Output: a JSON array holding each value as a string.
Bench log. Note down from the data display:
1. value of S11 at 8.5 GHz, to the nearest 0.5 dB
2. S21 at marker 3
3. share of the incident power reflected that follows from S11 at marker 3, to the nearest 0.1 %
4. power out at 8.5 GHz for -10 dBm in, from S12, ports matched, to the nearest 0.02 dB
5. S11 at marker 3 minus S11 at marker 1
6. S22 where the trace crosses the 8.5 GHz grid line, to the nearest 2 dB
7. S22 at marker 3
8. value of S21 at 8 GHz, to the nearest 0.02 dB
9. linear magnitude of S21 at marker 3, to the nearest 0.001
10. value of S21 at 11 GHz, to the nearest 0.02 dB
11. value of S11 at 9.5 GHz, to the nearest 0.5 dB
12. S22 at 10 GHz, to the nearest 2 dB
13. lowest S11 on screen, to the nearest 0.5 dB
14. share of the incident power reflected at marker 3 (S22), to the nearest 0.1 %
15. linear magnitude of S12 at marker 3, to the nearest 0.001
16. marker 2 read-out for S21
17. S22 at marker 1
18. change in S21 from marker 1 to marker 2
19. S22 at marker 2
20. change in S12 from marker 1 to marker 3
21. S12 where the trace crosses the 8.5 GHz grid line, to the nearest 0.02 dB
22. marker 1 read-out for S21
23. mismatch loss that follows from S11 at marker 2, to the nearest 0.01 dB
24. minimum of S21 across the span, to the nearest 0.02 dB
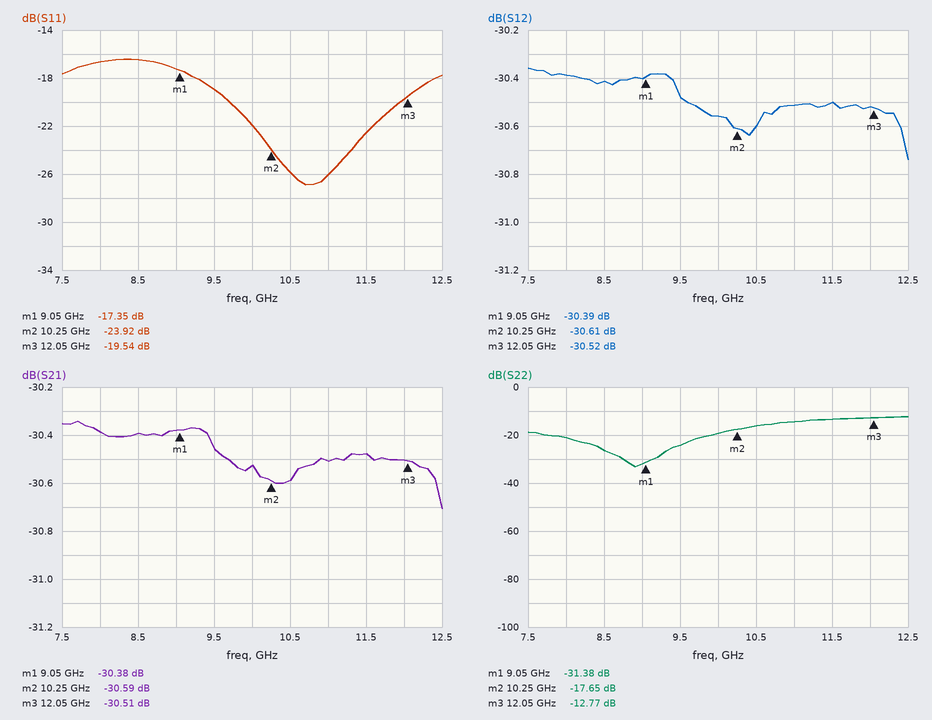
["-16.5 dB", "-30.51 dB", "1.1 %", "-40.42 dBm", "-2.19 dB", "-26 dB", "-12.77 dB", "-30.38 dB", "0.030", "-30.50 dB", "-19.0 dB", "-20 dB", "-27.0 dB", "5.3 %", "0.030", "-30.59 dB", "-31.38 dB", "-0.21 dB", "-17.65 dB", "-0.13 dB", "-30.42 dB", "-30.38 dB", "0.02 dB", "-30.70 dB"]
